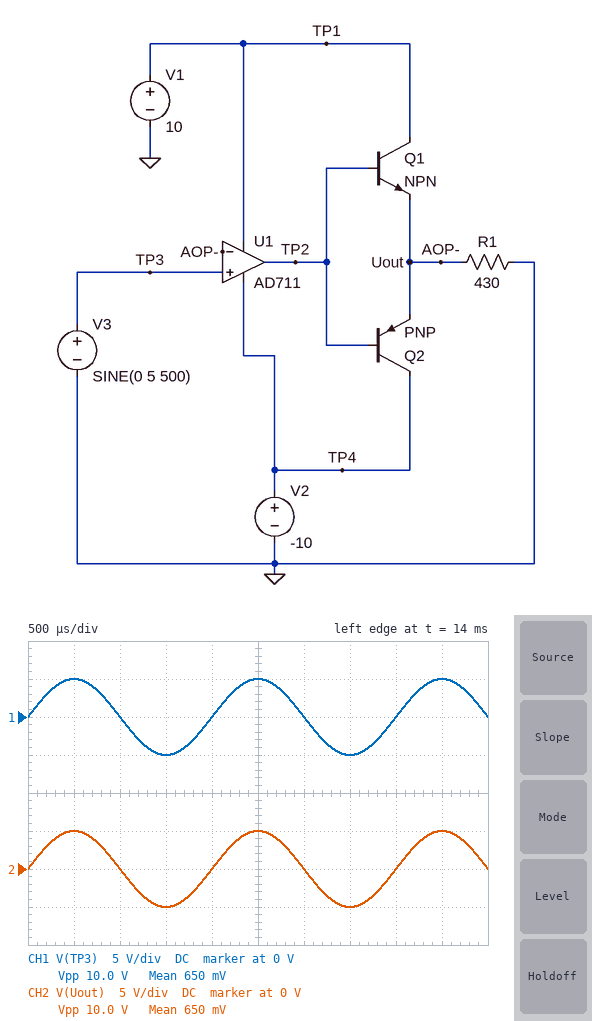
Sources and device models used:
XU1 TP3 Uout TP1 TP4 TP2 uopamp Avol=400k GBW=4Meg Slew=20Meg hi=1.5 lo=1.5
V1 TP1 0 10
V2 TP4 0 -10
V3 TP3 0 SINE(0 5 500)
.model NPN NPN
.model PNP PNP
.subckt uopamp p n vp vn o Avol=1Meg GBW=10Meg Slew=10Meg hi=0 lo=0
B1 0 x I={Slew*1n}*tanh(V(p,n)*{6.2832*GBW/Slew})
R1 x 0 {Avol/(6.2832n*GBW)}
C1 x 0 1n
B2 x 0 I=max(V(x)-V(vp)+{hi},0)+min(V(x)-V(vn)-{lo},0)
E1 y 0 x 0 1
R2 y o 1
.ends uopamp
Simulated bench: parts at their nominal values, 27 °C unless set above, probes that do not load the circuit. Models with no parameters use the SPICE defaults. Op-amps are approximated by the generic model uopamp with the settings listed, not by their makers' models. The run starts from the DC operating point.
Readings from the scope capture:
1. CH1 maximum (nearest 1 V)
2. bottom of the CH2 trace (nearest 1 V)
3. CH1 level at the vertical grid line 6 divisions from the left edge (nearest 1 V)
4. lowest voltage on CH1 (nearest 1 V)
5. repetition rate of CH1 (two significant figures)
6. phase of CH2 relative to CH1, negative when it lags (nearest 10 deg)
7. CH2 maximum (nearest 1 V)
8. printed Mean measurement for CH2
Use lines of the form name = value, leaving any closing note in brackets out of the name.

CH1 maximum = 5 V
bottom of the CH2 trace = -5 V
CH1 level at the vertical grid line 6 divisions from the left edge = 0 V
lowest voltage on CH1 = -5 V
repetition rate of CH1 = 500 Hz
phase of CH2 relative to CH1, negative when it lags = 0 deg
CH2 maximum = 5 V
printed Mean measurement for CH2 = 650 mV
